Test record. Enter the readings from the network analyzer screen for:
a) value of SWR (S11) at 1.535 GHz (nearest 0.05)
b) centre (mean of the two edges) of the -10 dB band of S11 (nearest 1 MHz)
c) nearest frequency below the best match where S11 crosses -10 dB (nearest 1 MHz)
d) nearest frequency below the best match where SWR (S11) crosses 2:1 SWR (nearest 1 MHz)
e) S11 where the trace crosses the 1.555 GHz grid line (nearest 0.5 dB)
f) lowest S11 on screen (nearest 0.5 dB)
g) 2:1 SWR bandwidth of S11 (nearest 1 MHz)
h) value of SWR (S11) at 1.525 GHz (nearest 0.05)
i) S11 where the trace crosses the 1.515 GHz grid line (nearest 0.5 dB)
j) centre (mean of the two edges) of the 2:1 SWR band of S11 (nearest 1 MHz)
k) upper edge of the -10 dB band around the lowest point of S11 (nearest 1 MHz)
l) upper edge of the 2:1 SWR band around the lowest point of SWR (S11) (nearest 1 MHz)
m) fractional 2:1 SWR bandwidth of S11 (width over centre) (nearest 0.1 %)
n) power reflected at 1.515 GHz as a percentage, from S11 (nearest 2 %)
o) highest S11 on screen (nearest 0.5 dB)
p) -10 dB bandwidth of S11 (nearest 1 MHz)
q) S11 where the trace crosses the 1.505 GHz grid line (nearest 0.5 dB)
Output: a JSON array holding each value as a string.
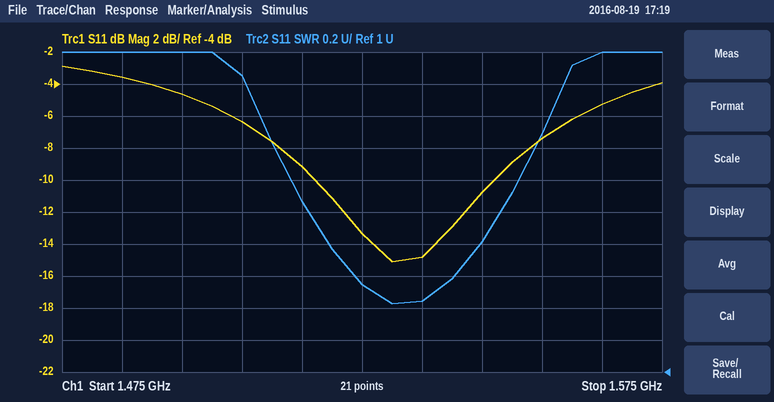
["1.45", "1.532 GHz", "1.517 GHz", "1.516 GHz", "-7.5 dB", "-15.0 dB", "32 MHz", "1.55", "-9.0 dB", "1.532 GHz", "1.547 GHz", "1.548 GHz", "2.1 %", "12 %", "-3.0 dB", "30 MHz", "-6.5 dB"]
